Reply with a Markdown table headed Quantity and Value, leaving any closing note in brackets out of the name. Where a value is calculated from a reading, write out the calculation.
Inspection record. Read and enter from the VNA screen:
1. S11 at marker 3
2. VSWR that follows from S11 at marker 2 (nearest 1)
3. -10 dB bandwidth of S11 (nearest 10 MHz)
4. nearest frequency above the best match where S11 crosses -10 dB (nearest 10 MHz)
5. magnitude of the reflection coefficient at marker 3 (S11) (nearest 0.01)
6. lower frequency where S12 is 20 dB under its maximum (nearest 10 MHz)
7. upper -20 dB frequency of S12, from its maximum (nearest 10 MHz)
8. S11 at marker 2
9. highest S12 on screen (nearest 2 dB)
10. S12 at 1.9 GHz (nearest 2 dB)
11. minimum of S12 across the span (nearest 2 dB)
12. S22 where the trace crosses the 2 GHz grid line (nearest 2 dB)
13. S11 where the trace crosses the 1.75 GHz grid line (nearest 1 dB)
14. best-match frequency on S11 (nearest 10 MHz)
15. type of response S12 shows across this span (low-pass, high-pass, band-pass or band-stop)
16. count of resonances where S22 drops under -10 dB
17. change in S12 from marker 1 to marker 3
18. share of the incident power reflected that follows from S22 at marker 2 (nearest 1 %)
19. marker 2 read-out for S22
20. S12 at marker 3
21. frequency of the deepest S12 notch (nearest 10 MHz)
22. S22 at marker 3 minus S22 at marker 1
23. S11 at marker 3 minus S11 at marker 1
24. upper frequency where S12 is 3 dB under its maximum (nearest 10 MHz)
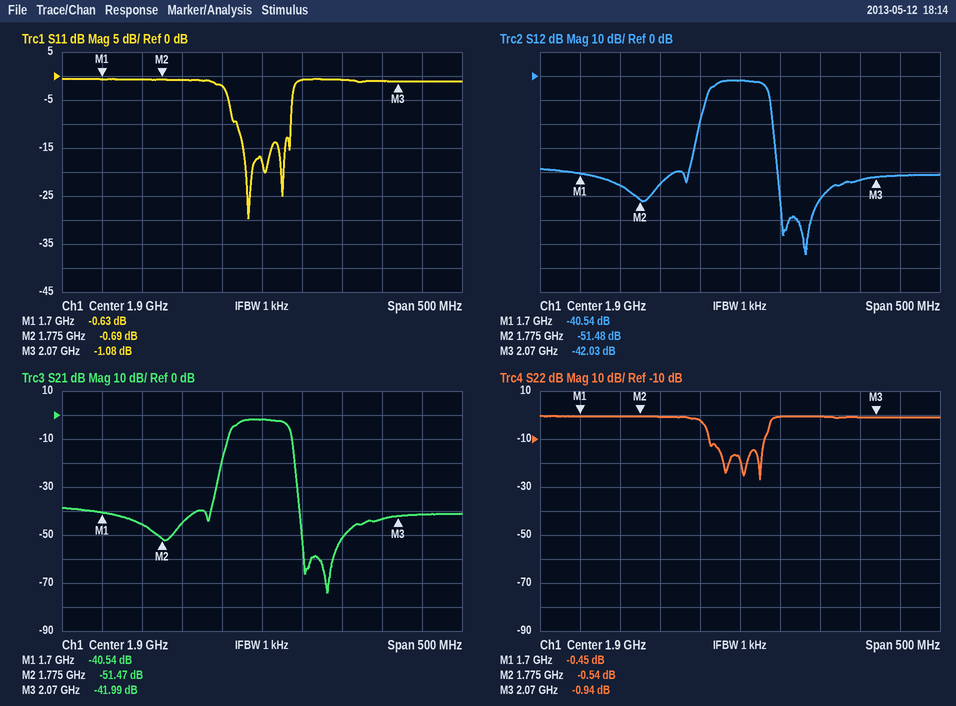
| Quantity | Value |
|---|---|
| S11 at marker 3 | -1.08 dB |
| VSWR that follows from S11 at marker 2 | (1 + 0.9236)/(1 − 0.9236) ≈ 25 |
| -10 dB bandwidth of S11 | 1.94 GHz − 1.87 GHz = 70 MHz |
| nearest frequency above the best match where S11 crosses -10 dB | 1.94 GHz |
| magnitude of the reflection coefficient at marker 3 (S11) | 10^(-1.08/20) ≈ 0.88 |
| lower frequency where S12 is 20 dB under its maximum | 1.85 GHz |
| upper -20 dB frequency of S12, from its maximum | 1.94 GHz |
| S11 at marker 2 | -0.69 dB |
| highest S12 on screen | -2 dB |
| S12 at 1.9 GHz | -2 dB |
| minimum of S12 across the span | -74 dB |
| S22 where the trace crosses the 2 GHz grid line | 0 dB |
| S11 where the trace crosses the 1.75 GHz grid line | -1 dB |
| best-match frequency on S11 | 1.88 GHz |
| type of response S12 shows across this span | band-pass |
| count of resonances where S22 drops under -10 dB | 3 |
| change in S12 from marker 1 to marker 3 | -42.03 − (-40.54) = -1.49 dB |
| share of the incident power reflected that follows from S22 at marker 2 | 10^(-0.54/10) ≈ 88 % |
| marker 2 read-out for S22 | -0.54 dB |
| S12 at marker 3 | -42.03 dB |
| frequency of the deepest S12 notch | 1.98 GHz |
| S22 at marker 3 minus S22 at marker 1 | -0.94 − (-0.45) = -0.49 dB |
| S11 at marker 3 minus S11 at marker 1 | -1.08 − (-0.63) = -0.45 dB |
| upper frequency where S12 is 3 dB under its maximum | 1.93 GHz |
